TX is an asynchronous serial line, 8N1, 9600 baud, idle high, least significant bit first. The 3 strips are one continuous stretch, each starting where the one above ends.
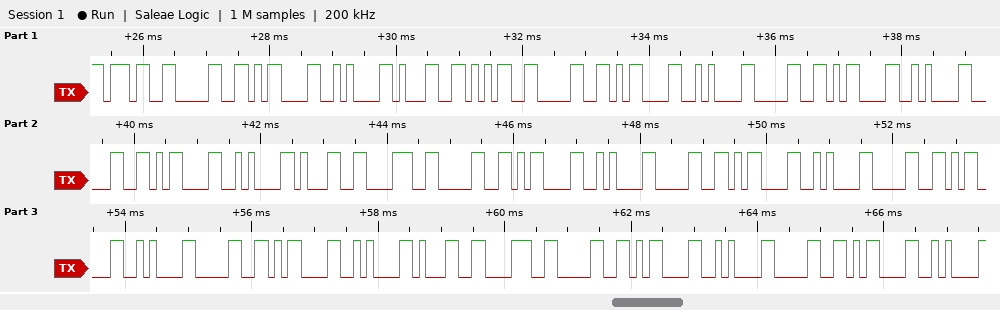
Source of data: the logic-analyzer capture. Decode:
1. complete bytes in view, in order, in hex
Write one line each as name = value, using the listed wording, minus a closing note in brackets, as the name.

complete bytes in view, in order, in hex = 37 30 0D 0A 31 35 30 0D 0A 30 0D 0A 30 0D 0A 31 38 30 0D 0A 30 0D 0A 30 0D 0A 30 0D 0A 31 38 30 0D 0A 30 0D 0A
